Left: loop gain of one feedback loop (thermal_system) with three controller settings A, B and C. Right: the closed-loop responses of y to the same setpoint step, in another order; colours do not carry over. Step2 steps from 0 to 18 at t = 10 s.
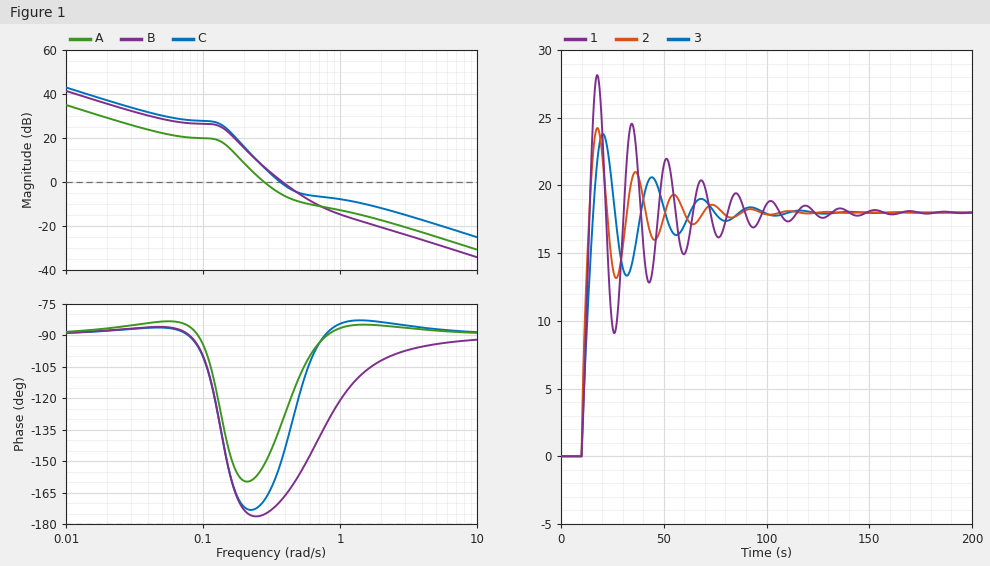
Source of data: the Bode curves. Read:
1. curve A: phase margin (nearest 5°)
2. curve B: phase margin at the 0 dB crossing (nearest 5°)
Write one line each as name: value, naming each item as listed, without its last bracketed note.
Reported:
curve A: phase margin: 30°
curve B: phase margin at the 0 dB crossing: 10°
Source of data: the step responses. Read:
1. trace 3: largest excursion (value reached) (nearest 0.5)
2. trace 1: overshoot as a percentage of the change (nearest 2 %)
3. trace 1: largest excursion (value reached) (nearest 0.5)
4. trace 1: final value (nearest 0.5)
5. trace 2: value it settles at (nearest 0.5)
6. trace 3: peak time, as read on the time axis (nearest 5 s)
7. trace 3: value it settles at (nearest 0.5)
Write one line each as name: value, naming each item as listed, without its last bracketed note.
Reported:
trace 3: largest excursion (value reached): 24.0
trace 1: overshoot as a percentage of the change: 56 %
trace 1: largest excursion (value reached): 28.0
trace 1: final value: 18.0
trace 2: value it settles at: 18.0
trace 3: peak time, as read on the time axis: 20 s
trace 3: value it settles at: 18.0
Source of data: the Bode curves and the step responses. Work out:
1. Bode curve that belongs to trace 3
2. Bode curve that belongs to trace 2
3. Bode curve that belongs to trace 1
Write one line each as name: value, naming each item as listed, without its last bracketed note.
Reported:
Bode curve that belongs to trace 3: A
Bode curve that belongs to trace 2: C
Bode curve that belongs to trace 1: B
